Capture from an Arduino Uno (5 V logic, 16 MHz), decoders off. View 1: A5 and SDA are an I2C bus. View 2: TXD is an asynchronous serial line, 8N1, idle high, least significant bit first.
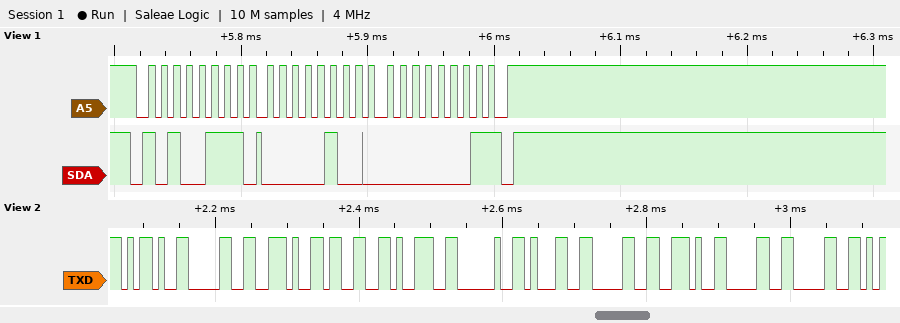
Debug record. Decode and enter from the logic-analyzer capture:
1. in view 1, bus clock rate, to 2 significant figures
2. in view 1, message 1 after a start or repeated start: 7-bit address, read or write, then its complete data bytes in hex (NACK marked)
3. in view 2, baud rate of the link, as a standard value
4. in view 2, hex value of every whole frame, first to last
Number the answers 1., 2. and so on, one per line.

1. 100 kHz
2. 0x53 read: 04 01 NACK
3. 115200 baud
4. 2D 30 2E 33 39 20 31 30 2E 30 30
